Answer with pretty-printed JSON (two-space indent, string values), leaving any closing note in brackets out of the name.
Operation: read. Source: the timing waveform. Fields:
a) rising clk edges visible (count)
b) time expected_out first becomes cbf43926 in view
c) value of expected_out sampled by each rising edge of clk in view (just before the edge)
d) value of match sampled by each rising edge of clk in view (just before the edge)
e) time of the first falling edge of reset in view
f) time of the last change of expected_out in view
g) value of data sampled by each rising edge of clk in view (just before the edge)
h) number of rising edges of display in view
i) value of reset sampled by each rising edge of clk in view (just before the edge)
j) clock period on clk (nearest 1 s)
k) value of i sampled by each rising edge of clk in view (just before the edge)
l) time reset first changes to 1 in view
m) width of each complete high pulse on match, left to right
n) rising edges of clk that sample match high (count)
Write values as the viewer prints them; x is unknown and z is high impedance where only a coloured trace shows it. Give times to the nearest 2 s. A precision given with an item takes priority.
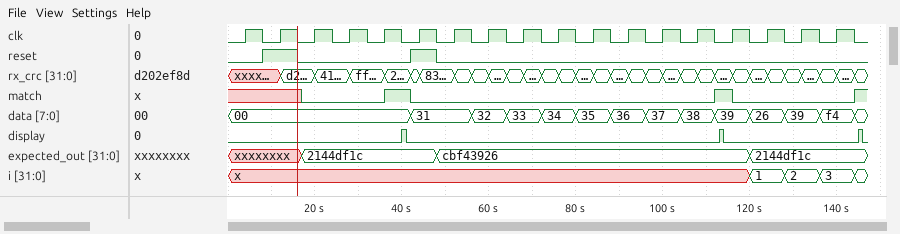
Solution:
{
  "rising clk edges visible": "18",
  "time expected_out first becomes cbf43926 in view": "48 s",
  "value of expected_out sampled by each rising edge of clk in view": "xxxxxxxx, xxxxxxxx, 2144df1c, 2144df1c, 2144df1c, 2144df1c, cbf43926, cbf43926, cbf43926, cbf43926, cbf43926, cbf43926, cbf43926, cbf43926, cbf43926, 2144df1c, 2144df1c, 2144df1c",
  "value of match sampled by each rising edge of clk in view": "x x 0 0 0 0 0 0 0 0 0 0 0 0 1 0 0 0",
  "time of the first falling edge of reset in view": "16 s",
  "time of the last change of expected_out in view": "120 s",
  "value of data sampled by each rising edge of clk in view": "00, 00, 00, 00, 00, 31, 31, 32, 33, 34, 35, 36, 37, 38, 39, 26, 39, f4",
  "number of rising edges of display in view": "3",
  "value of reset sampled by each rising edge of clk in view": "0 1 0 0 0 1 0 0 0 0 0 0 0 0 0 0 0 0",
  "clock period on clk": "8 s",
  "value of i sampled by each rising edge of clk in view": "x, x, x, x, x, x, x, x, x, x, x, x, x, x, x, 1, 2, 3",
  "time reset first changes to 1 in view": "8 s",
  "width of each complete high pulse on match, left to right": "6 s, 4 s",
  "rising edges of clk that sample match high": "1"
}
